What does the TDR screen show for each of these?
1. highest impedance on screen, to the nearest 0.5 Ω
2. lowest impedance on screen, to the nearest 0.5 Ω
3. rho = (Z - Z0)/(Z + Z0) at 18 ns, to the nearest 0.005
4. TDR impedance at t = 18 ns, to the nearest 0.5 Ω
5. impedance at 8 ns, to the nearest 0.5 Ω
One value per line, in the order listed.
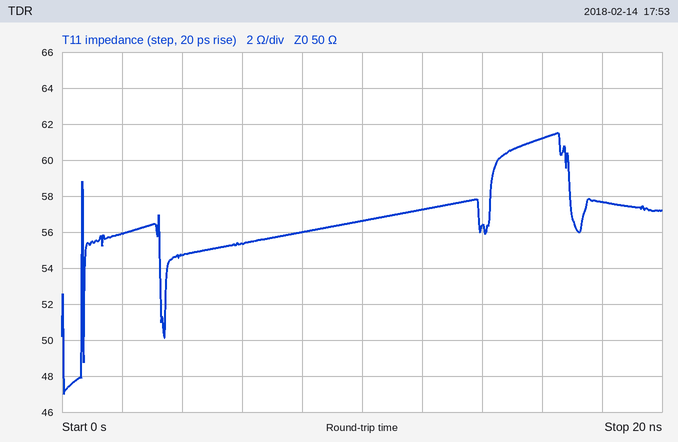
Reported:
61.5 Ω
47.0 Ω
+0.070
57.5 Ω
56.0 Ω
